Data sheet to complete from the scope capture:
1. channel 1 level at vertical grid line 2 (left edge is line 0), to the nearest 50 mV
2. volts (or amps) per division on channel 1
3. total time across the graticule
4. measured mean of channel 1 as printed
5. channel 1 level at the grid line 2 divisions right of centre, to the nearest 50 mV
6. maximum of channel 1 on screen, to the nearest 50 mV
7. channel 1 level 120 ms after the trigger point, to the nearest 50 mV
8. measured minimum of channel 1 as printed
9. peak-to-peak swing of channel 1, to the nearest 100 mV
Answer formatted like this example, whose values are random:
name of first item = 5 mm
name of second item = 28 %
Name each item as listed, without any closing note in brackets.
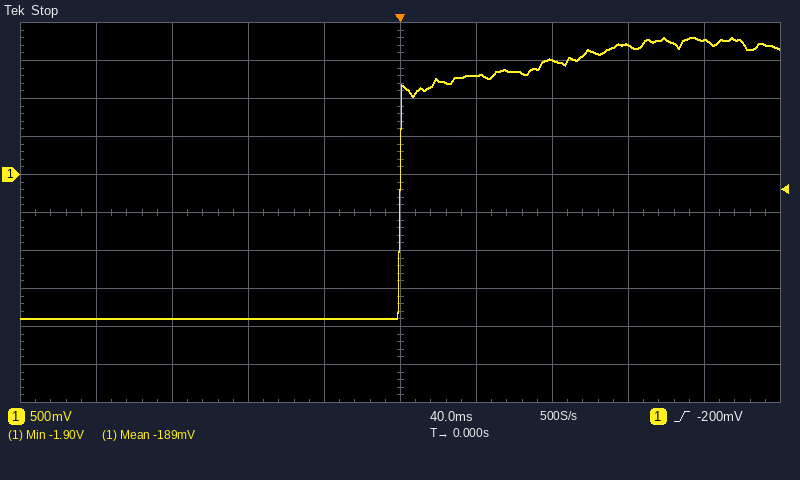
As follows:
channel 1 level at vertical grid line 2 (left edge is line 0), to the nearest 50 mV = -1.90 V
volts (or amps) per division on channel 1 = 500 mV
total time across the graticule = 400 ms
measured mean of channel 1 as printed = -189 mV
channel 1 level at the grid line 2 divisions right of centre, to the nearest 50 mV = 1.50 V
maximum of channel 1 on screen, to the nearest 50 mV = 1.80 V
channel 1 level 120 ms after the trigger point, to the nearest 50 mV = 1.70 V
measured minimum of channel 1 as printed = -1.90 V
peak-to-peak swing of channel 1, to the nearest 100 mV = 3.70 V
